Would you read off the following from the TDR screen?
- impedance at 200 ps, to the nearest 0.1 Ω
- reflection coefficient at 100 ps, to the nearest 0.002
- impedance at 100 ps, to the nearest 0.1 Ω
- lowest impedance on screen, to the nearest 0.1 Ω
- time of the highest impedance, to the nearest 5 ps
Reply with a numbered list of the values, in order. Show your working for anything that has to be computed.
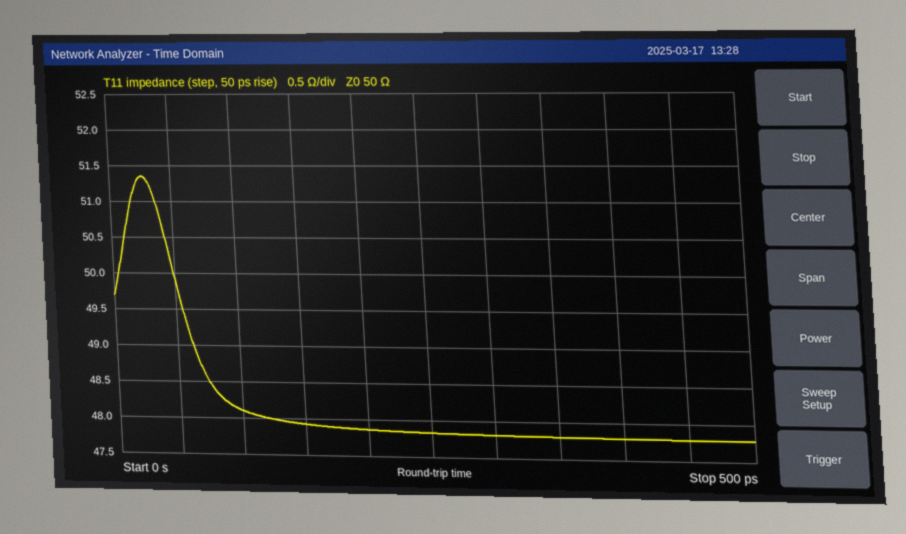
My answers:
1. 47.9 Ω
2. (48.1 − 50)/(48.1 + 50) ≈ -0.0194, so -0.020 to the nearest 0.002
3. 48.1 Ω
4. 47.8 Ω
5. 25 ps
